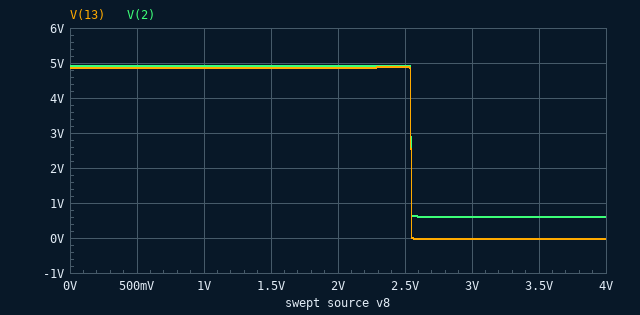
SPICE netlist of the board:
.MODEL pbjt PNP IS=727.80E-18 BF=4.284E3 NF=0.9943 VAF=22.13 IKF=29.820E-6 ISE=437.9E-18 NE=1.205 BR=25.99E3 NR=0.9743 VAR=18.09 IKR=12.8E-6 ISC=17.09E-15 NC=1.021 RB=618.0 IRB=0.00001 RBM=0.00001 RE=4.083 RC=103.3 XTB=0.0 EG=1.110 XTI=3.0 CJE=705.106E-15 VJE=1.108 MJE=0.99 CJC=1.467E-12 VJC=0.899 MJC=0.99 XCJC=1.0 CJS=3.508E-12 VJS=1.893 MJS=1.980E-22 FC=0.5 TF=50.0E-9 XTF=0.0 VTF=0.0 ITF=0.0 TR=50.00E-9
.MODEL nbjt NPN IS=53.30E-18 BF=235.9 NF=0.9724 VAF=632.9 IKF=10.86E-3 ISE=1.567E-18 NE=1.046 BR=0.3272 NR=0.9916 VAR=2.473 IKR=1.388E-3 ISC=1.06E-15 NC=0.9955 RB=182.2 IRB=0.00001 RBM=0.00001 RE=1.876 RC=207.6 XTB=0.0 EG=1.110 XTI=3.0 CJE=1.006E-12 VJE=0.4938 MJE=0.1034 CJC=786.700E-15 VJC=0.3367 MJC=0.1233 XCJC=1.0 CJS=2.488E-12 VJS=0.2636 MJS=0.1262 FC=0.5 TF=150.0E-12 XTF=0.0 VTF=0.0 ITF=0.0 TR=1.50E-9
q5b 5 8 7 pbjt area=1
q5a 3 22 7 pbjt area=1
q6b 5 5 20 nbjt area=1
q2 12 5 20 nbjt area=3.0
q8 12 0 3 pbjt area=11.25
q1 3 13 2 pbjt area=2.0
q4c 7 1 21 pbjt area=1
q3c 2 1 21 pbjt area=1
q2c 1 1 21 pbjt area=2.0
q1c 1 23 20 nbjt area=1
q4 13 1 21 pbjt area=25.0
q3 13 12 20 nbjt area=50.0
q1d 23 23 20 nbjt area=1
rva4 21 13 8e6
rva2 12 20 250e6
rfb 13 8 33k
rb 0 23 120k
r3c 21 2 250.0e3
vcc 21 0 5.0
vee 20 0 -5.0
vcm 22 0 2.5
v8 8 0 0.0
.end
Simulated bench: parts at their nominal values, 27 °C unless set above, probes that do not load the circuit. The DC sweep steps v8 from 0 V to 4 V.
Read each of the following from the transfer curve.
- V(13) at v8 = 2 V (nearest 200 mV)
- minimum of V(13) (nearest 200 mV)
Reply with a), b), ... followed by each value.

a) 4.8 V
b) 0 V
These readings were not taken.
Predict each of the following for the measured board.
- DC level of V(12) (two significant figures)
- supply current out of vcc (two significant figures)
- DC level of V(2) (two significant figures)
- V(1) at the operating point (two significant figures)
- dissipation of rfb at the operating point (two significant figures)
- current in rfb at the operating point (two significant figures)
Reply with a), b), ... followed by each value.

a) -4.9 V
b) 190 µA
c) 4.9 V
d) 4.4 V
e) 710 µW
f) 150 µA
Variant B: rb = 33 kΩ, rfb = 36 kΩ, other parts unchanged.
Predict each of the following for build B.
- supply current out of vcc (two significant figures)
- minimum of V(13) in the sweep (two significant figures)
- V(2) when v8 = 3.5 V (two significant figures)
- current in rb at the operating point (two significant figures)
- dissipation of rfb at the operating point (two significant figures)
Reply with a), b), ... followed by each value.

a) 280 µA
b) -35 mV
c) 640 mV
d) 130 µA
e) 660 µW
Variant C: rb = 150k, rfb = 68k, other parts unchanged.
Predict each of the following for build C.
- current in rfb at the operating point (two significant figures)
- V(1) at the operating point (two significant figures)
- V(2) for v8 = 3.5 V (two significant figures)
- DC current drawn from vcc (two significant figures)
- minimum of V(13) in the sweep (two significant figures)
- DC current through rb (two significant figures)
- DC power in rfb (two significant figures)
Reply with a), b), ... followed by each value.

a) 72 µA
b) 4.4 V
c) 600 mV
d) 110 µA
e) -37 mV
f) 29 µA
g) 350 µW
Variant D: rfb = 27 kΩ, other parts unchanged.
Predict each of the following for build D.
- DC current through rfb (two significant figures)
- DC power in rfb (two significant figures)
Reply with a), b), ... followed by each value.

a) 180 µA
b) 870 µW
